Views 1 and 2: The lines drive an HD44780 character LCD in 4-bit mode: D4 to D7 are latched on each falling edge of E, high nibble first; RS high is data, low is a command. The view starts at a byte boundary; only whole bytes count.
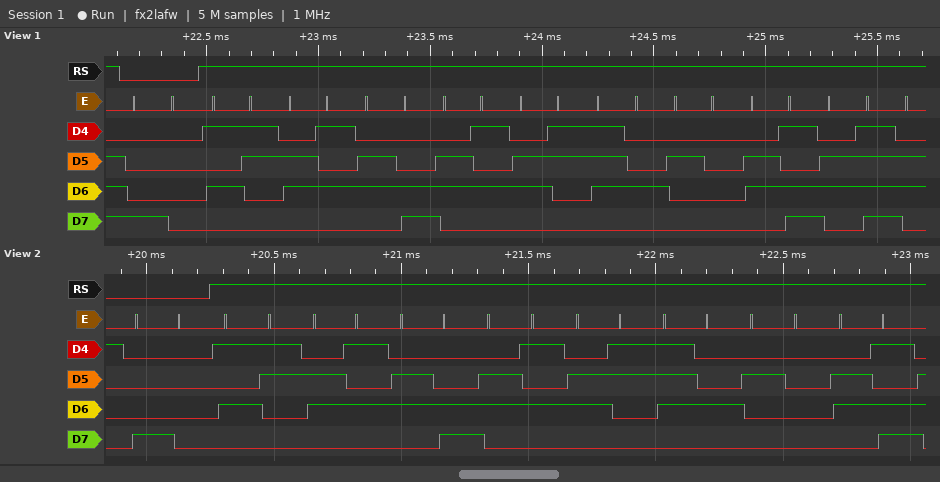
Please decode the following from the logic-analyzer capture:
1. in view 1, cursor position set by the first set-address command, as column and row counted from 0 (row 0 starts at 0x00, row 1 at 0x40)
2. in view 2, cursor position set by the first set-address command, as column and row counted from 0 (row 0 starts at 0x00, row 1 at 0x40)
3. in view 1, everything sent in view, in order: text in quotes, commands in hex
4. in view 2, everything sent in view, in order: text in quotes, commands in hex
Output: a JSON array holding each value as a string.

["column 0, row 0", "column 0, row 0", "0x80 \"Select mo\"", "0x80 \"Select m\""]
